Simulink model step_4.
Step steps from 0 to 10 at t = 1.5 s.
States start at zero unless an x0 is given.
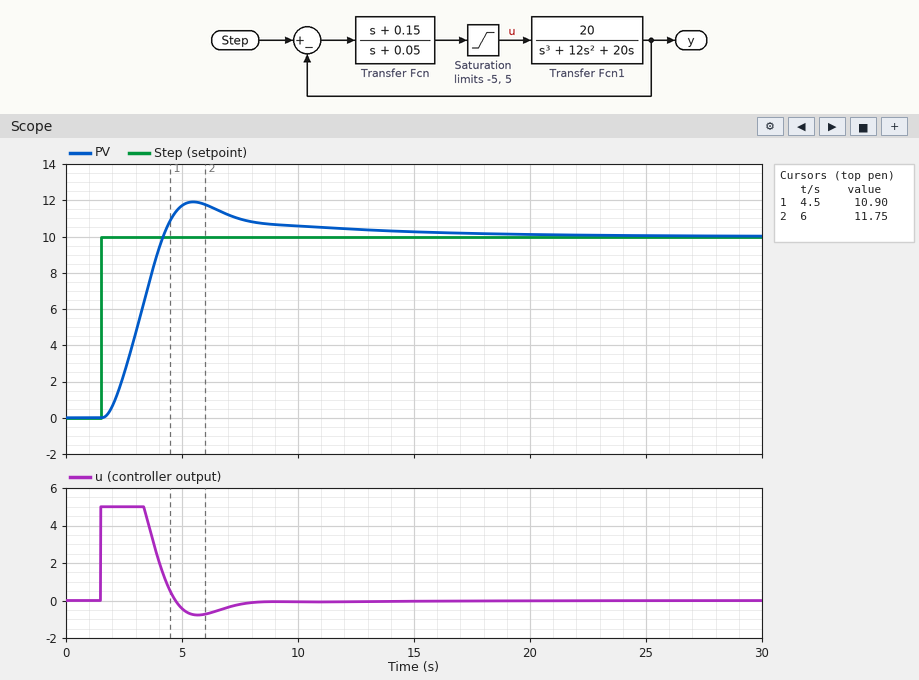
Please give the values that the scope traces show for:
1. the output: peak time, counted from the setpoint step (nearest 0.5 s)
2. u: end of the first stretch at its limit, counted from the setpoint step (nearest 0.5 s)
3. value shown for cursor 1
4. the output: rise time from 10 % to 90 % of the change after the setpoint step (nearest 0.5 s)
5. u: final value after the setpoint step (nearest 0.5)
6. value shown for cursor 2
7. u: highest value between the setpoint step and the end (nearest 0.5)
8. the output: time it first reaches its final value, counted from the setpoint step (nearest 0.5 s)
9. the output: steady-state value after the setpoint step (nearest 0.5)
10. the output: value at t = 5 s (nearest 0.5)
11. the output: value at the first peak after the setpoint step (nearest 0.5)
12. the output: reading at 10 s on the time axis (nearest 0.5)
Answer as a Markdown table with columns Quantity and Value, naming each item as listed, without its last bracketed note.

| Quantity | Value |
|---|---|
| the output: peak time, counted from the setpoint step | 4.0 s |
| u: end of the first stretch at its limit, counted from the setpoint step | 2.0 s |
| value shown for cursor 1 | 10.90 |
| the output: rise time from 10 % to 90 % of the change after the setpoint step | 2.0 s |
| u: final value after the setpoint step | 0.0 |
| value shown for cursor 2 | 11.75 |
| u: highest value between the setpoint step and the end | 5.0 |
| the output: time it first reaches its final value, counted from the setpoint step | 2.5 s |
| the output: steady-state value after the setpoint step | 10.0 |
| the output: value at t = 5 s | 11.5 |
| the output: value at the first peak after the setpoint step | 12.0 |
| the output: reading at 10 s on the time axis | 10.5 |
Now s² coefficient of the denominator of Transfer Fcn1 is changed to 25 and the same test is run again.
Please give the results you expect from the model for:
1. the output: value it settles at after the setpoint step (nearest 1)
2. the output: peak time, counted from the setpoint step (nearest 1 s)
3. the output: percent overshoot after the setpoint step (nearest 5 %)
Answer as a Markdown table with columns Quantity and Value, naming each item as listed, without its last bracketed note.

| Quantity | Value |
|---|---|
| the output: value it settles at after the setpoint step | 10 |
| the output: peak time, counted from the setpoint step | 5 s |
| the output: percent overshoot after the setpoint step | 35 % |
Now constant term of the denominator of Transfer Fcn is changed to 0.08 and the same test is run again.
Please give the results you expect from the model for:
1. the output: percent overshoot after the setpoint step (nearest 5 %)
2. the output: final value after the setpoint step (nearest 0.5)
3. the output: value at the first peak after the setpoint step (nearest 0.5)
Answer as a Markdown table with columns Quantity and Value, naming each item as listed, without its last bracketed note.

| Quantity | Value |
|---|---|
| the output: percent overshoot after the setpoint step | 15 % |
| the output: final value after the setpoint step | 10.0 |
| the output: value at the first peak after the setpoint step | 11.5 |
